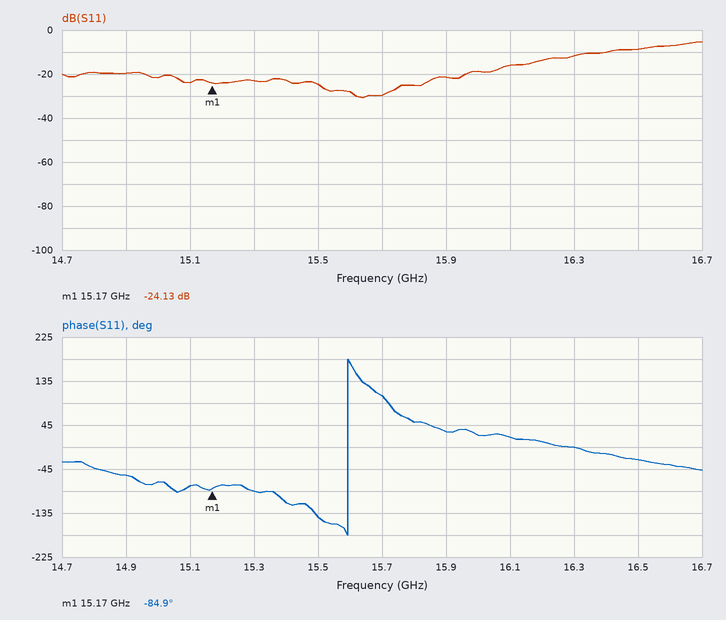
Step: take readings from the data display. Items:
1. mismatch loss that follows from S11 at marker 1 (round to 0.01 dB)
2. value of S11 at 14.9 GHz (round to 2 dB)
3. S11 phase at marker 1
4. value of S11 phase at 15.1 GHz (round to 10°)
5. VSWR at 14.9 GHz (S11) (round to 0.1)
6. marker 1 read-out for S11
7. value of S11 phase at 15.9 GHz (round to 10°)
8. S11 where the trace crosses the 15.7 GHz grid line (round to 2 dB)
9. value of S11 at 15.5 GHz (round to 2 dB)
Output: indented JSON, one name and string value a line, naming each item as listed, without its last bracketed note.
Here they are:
{
  "mismatch loss that follows from S11 at marker 1": "0.02 dB",
  "value of S11 at 14.9 GHz": "-20 dB",
  "S11 phase at marker 1": "-84.9°",
  "value of S11 phase at 15.1 GHz": "-80°",
  "VSWR at 14.9 GHz (S11)": "1.2",
  "marker 1 read-out for S11": "-24.13 dB",
  "value of S11 phase at 15.9 GHz": "30°",
  "S11 where the trace crosses the 15.7 GHz grid line": "-30 dB",
  "value of S11 at 15.5 GHz": "-24 dB"
}
